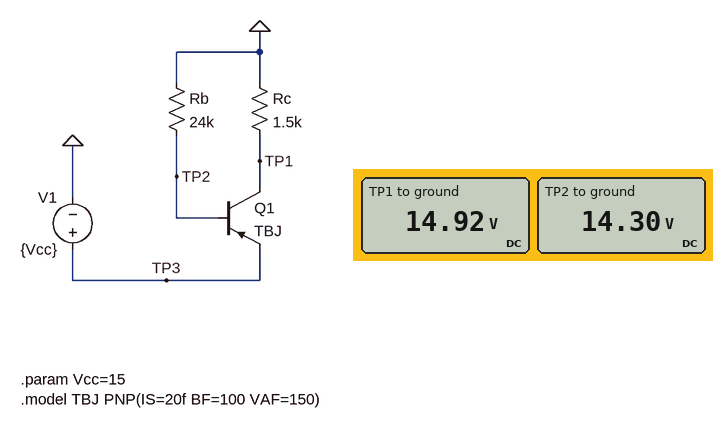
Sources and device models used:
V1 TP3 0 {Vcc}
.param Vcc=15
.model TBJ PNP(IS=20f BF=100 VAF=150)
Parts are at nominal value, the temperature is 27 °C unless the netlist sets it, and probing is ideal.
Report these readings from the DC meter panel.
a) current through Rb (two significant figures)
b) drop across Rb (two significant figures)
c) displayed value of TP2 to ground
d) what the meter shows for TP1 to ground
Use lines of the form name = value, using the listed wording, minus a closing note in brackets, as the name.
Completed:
current through Rb = 600 µA
drop across Rb = 14 V
displayed value of TP2 to ground = 14.30 V
what the meter shows for TP1 to ground = 14.92 V
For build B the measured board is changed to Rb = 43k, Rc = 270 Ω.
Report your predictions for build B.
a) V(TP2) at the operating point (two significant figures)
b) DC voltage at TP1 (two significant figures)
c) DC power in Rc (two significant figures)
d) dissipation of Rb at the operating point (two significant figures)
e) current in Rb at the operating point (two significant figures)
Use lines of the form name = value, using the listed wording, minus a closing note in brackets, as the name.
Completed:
V(TP2) at the operating point = 14 V
DC voltage at TP1 = 9.3 V
DC power in Rc = 320 mW
dissipation of Rb at the operating point = 4.7 mW
current in Rb at the operating point = 330 µA
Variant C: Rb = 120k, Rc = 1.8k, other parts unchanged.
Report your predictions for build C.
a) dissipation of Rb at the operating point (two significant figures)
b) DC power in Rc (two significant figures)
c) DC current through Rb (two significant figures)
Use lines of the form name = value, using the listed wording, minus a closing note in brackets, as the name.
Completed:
dissipation of Rb at the operating point = 1.7 mW
DC power in Rc = 120 mW
DC current through Rb = 120 µA
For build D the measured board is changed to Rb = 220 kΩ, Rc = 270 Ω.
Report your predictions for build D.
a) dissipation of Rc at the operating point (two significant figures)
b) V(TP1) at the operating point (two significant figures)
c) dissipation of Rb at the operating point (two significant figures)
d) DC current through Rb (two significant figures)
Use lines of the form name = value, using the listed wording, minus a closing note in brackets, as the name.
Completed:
dissipation of Rc at the operating point = 13 mW
V(TP1) at the operating point = 1.9 V
dissipation of Rb at the operating point = 930 µW
DC current through Rb = 65 µA
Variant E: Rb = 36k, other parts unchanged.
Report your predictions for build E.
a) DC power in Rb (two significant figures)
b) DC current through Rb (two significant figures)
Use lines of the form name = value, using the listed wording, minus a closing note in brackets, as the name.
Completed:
DC power in Rb = 5.7 mW
DC current through Rb = 400 µA
